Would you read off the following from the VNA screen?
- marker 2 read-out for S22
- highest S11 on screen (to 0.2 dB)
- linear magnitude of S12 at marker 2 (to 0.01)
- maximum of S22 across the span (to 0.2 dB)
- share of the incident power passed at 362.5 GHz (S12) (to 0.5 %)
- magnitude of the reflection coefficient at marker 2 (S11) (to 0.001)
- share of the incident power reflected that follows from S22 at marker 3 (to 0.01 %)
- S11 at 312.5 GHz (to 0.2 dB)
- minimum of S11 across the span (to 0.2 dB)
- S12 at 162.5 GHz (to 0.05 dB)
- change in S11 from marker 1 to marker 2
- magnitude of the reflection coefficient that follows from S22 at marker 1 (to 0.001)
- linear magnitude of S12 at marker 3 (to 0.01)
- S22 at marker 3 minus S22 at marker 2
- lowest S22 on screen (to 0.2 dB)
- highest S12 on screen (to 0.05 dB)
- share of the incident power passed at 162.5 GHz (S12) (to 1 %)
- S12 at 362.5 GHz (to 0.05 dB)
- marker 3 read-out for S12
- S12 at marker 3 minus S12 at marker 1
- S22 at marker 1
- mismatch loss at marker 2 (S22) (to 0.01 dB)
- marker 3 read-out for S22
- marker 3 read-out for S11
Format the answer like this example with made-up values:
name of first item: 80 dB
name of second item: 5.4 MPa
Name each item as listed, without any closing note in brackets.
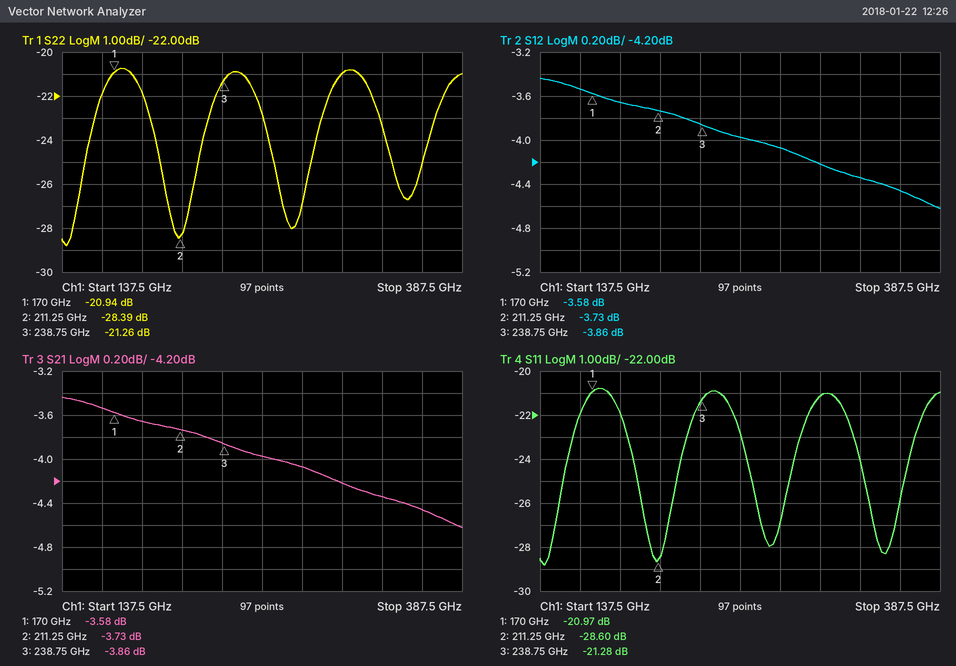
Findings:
marker 2 read-out for S22: -28.39 dB
highest S11 on screen: -20.8 dB
linear magnitude of S12 at marker 2: 0.65
maximum of S22 across the span: -20.8 dB
share of the incident power passed at 362.5 GHz (S12): 36.0 %
magnitude of the reflection coefficient at marker 2 (S11): 0.037
share of the incident power reflected that follows from S22 at marker 3: 0.75 %
S11 at 312.5 GHz: -21.2 dB
minimum of S11 across the span: -28.8 dB
S12 at 162.5 GHz: -3.55 dB
change in S11 from marker 1 to marker 2: -7.63 dB
magnitude of the reflection coefficient that follows from S22 at marker 1: 0.090
linear magnitude of S12 at marker 3: 0.64
S22 at marker 3 minus S22 at marker 2: 7.13 dB
lowest S22 on screen: -28.8 dB
highest S12 on screen: -3.45 dB
share of the incident power passed at 162.5 GHz (S12): 44 %
S12 at 362.5 GHz: -4.45 dB
marker 3 read-out for S12: -3.86 dB
S12 at marker 3 minus S12 at marker 1: -0.28 dB
S22 at marker 1: -20.94 dB
mismatch loss at marker 2 (S22): 0.01 dB
marker 3 read-out for S22: -21.26 dB
marker 3 read-out for S11: -21.28 dB
